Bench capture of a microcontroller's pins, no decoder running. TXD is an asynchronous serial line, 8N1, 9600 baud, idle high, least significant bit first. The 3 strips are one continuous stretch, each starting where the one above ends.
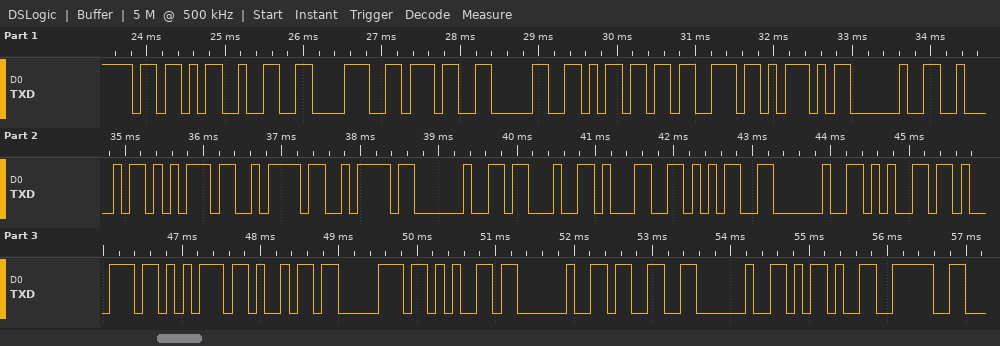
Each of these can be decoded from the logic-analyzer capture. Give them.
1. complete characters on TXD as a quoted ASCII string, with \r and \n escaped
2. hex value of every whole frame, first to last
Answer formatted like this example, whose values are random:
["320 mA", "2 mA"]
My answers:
["\"[2870ms] Buzz #15 equipe 3 ->\"", "5B 32 38 37 30 6D 73 5D 20 42 75 7A 7A 20 23 31 35 20 65 71 75 69 70 65 20 33 20 2D 3E"]
